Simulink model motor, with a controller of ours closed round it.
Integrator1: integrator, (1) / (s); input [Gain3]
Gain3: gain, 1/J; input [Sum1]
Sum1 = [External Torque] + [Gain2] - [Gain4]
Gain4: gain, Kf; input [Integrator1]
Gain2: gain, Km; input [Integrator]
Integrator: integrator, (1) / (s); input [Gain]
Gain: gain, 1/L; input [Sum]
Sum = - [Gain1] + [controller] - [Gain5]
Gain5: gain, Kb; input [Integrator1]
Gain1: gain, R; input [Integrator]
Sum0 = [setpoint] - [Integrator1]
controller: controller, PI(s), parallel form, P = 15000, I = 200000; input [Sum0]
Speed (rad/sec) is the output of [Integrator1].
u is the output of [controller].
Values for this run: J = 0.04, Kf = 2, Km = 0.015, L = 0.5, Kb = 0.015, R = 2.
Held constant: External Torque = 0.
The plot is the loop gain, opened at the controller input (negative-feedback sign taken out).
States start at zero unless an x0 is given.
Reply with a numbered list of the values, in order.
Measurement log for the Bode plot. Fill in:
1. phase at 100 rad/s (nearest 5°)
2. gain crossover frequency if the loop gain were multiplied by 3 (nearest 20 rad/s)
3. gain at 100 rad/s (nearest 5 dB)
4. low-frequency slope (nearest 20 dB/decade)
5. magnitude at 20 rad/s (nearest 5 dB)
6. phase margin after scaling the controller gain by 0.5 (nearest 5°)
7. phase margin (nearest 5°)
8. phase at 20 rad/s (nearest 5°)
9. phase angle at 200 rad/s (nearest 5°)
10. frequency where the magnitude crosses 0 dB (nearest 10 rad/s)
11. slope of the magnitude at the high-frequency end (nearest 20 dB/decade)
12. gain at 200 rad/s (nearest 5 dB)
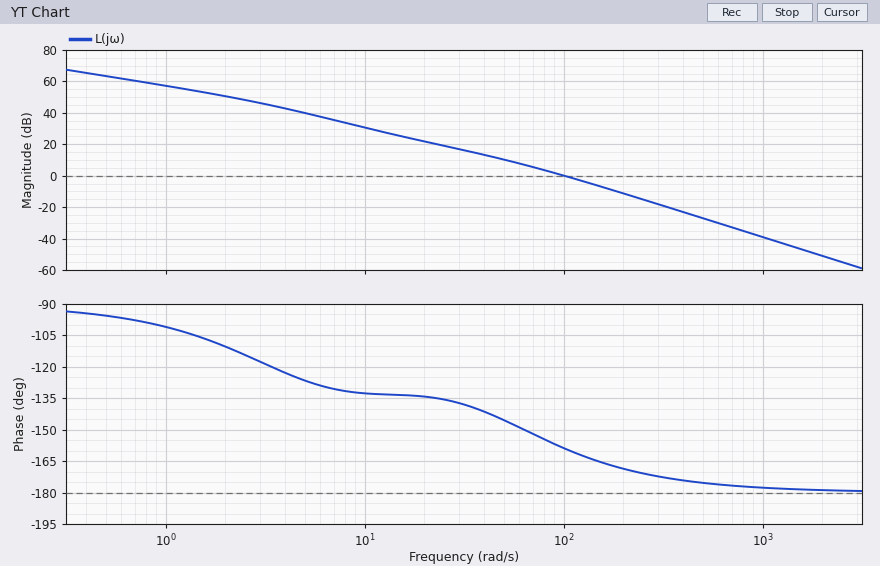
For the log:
1. -160°
2. 180 rad/s
3. 0 dB
4. -20 dB/decade
5. 20 dB
6. 30°
7. 20°
8. -135°
9. -170°
10. 100 rad/s
11. -40 dB/decade
12. -10 dB
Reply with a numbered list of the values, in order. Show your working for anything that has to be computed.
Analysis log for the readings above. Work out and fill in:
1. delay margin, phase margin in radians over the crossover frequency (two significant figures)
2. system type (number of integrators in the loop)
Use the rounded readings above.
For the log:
1. 20 × π / 180 / 100 = 0.0035 s
2. 1
